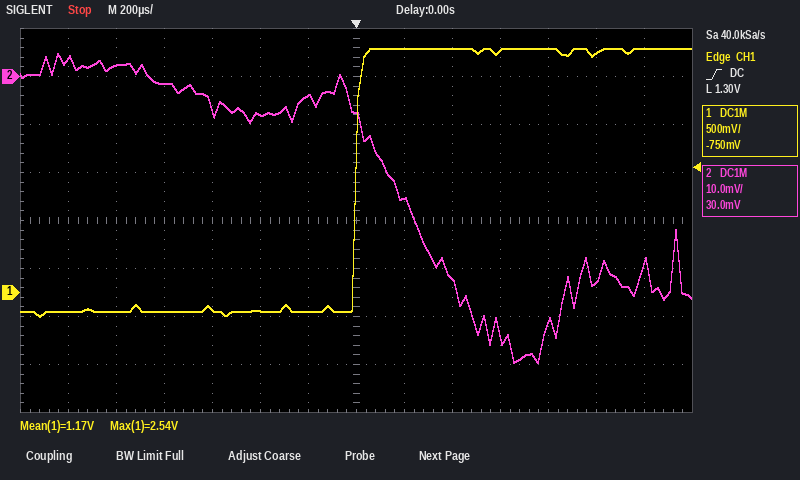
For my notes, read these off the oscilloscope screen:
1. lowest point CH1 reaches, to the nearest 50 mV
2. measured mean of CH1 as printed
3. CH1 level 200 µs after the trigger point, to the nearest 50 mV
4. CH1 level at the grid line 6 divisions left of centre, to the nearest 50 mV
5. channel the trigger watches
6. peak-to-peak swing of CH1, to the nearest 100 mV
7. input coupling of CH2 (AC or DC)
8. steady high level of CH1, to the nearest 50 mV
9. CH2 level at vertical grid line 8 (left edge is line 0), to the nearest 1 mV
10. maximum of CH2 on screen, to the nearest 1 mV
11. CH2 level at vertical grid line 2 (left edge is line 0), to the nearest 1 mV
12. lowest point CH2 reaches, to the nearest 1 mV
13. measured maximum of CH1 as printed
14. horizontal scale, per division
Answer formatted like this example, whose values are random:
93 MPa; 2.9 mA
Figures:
-250 mV; 1.17 V; 2.55 V; -200 mV; CH1; 2.80 V; DC; 2.55 V; -25 mV; 5 mV; 2 mV; -60 mV; 2.54 V; 200 µs
